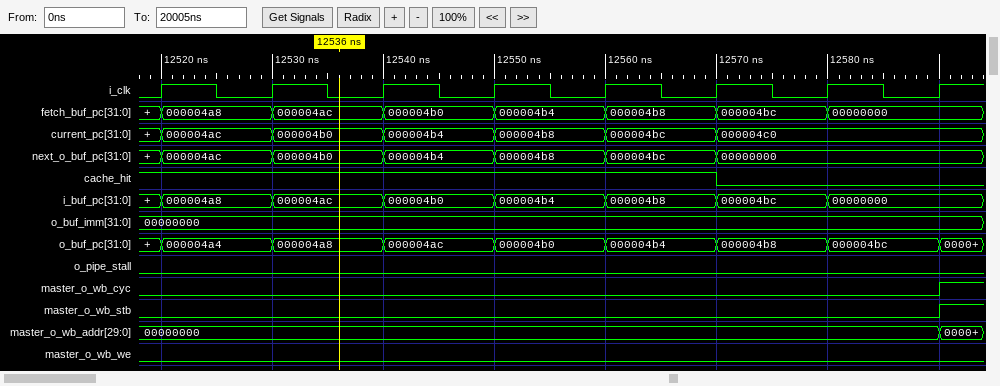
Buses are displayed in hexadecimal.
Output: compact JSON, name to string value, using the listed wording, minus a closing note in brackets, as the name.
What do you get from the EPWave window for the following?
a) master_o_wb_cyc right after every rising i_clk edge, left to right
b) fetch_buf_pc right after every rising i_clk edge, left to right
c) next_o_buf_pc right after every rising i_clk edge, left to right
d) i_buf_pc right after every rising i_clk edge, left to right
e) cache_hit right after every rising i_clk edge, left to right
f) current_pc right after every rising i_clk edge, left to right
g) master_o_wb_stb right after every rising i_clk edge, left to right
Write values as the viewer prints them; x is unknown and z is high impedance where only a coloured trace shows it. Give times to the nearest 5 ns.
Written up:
{"master_o_wb_cyc right after every rising i_clk edge, left to right": "0 0 0 0 0 0 0 1", "fetch_buf_pc right after every rising i_clk edge, left to right": "000004a8, 000004ac, 000004b0, 000004b4, 000004b8, 000004bc, 00000000, 00000000", "next_o_buf_pc right after every rising i_clk edge, left to right": "000004ac, 000004b0, 000004b4, 000004b8, 000004bc, 00000000, 00000000, 00000000", "i_buf_pc right after every rising i_clk edge, left to right": "000004a8, 000004ac, 000004b0, 000004b4, 000004b8, 000004bc, 00000000, 00000000", "cache_hit right after every rising i_clk edge, left to right": "1 1 1 1 1 0 0 0", "current_pc right after every rising i_clk edge, left to right": "000004ac, 000004b0, 000004b4, 000004b8, 000004bc, 000004c0, 000004c0, 000004c0", "master_o_wb_stb right after every rising i_clk edge, left to right": "0 0 0 0 0 0 0 1"}
